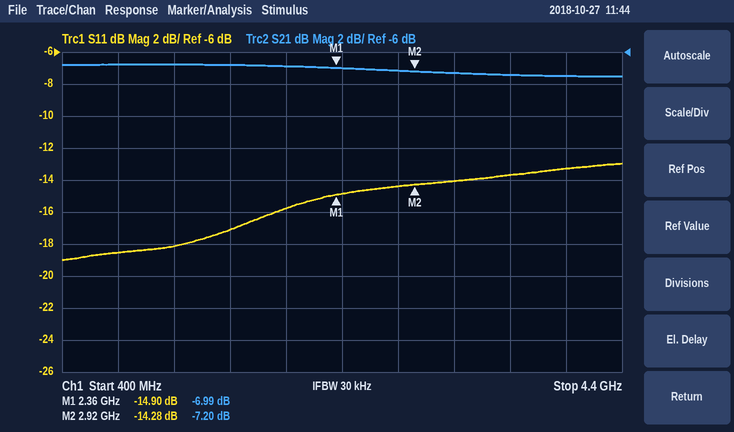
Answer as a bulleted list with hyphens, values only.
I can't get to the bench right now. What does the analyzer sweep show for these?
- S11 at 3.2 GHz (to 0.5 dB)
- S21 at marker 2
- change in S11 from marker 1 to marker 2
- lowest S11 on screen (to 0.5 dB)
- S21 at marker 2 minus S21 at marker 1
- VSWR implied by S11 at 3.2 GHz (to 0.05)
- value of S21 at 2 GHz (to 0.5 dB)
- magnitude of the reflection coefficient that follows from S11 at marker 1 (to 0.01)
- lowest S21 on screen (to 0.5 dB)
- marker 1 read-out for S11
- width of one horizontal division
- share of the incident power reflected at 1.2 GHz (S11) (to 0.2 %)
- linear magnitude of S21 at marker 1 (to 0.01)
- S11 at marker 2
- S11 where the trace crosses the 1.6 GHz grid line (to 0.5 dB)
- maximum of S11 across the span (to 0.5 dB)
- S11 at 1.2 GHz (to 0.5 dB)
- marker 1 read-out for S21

- -14.0 dB
- -7.20 dB
- 0.62 dB
- -19.0 dB
- -0.21 dB
- 1.50
- -7.0 dB
- 0.18
- -7.5 dB
- -14.90 dB
- 400 MHz
- 1.6 %
- 0.45
- -14.28 dB
- -17.0 dB
- -13.0 dB
- -18.0 dB
- -6.99 dB
